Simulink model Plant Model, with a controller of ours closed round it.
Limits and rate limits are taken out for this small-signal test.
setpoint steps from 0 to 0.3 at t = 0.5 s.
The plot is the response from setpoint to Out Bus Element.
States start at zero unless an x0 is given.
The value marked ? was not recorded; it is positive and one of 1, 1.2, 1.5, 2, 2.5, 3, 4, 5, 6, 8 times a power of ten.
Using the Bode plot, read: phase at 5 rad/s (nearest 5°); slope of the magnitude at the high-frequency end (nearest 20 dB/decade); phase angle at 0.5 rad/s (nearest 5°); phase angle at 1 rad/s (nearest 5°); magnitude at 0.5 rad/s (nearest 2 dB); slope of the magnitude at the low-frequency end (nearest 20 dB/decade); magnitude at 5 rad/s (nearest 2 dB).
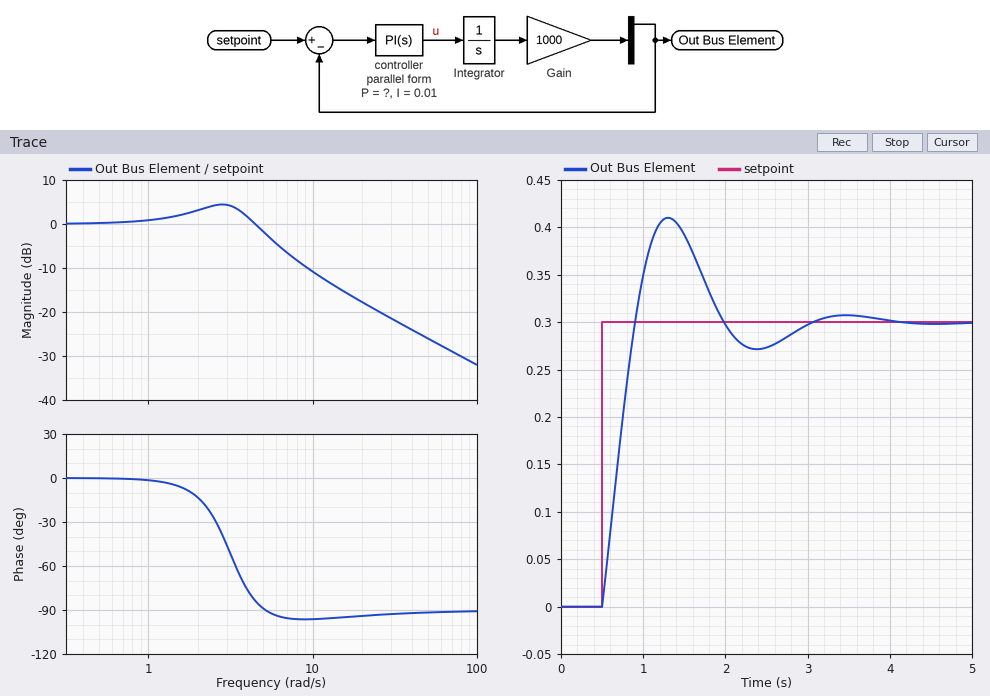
-90°
-20 dB/decade
0°
0°
0 dB
0 dB/decade
-2 dB
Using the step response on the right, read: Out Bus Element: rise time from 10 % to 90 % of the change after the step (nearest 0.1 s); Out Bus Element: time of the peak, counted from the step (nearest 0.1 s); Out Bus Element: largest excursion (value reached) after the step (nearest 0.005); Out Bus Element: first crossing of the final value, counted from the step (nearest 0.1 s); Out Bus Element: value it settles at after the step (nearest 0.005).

0.3 s
0.8 s
0.410
0.4 s
0.300
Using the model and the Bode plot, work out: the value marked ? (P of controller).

0.0025
